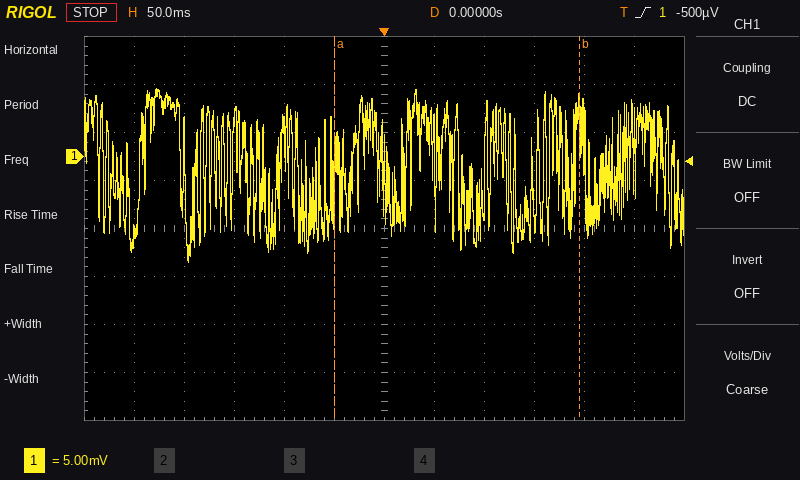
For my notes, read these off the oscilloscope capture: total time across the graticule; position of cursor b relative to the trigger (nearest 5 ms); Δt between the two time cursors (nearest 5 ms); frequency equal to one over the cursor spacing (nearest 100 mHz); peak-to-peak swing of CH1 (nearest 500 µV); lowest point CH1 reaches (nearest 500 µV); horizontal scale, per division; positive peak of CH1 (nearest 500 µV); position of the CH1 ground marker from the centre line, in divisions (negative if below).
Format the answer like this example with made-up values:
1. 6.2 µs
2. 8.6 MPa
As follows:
1. 600 ms
2. +195 ms
3. 245 ms
4. 4.1 Hz
5. 18.0 mV
6. -11.0 mV
7. 50 ms
8. 7.0 mV
9. +1.5 div
